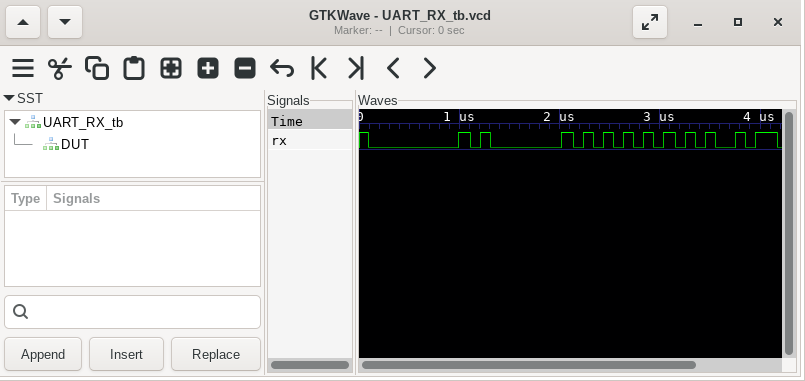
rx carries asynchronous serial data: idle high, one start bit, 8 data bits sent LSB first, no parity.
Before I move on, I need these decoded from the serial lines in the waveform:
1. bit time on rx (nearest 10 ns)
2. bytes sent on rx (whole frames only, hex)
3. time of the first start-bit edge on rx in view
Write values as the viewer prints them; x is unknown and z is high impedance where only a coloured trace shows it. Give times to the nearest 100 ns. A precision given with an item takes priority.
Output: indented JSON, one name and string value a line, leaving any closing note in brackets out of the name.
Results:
{
  "bit time on rx": "100 ns",
  "bytes sent on rx": "00, 01, 55, A5",
  "time of the first start-bit edge on rx in view": "100 ns"
}
